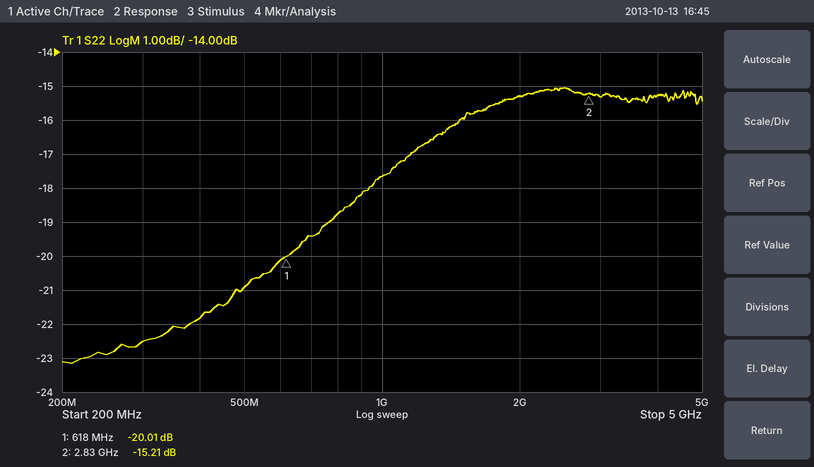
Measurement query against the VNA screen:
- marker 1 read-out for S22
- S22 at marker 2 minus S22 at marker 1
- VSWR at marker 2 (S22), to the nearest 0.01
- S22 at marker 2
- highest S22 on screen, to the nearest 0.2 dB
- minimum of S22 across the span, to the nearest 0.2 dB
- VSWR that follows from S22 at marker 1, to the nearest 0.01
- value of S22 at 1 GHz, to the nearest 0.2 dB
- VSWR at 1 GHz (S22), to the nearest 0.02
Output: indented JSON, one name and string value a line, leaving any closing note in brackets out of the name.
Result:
{
  "marker 1 read-out for S22": "-20.01 dB",
  "S22 at marker 2 minus S22 at marker 1": "4.80 dB",
  "VSWR at marker 2 (S22), to the nearest 0.01": "1.42",
  "S22 at marker 2": "-15.21 dB",
  "highest S22 on screen, to the nearest 0.2 dB": "-15.0 dB",
  "minimum of S22 across the span, to the nearest 0.2 dB": "-23.2 dB",
  "VSWR that follows from S22 at marker 1, to the nearest 0.01": "1.22",
  "value of S22 at 1 GHz, to the nearest 0.2 dB": "-17.6 dB",
  "VSWR at 1 GHz (S22), to the nearest 0.02": "1.30"
}
